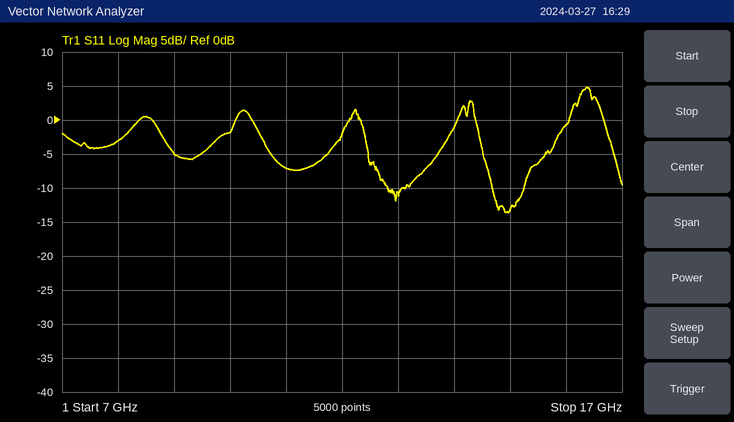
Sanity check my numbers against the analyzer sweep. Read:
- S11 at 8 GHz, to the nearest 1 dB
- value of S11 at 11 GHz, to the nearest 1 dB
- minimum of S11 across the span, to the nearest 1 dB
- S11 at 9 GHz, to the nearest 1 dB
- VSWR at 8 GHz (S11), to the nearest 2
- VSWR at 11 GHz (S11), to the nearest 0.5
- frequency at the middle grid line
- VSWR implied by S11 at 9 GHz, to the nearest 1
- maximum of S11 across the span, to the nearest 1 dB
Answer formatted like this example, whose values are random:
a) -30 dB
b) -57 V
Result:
a) -3 dB
b) -7 dB
c) -14 dB
d) -5 dB
e) 6
f) 2.5
g) 12 GHz
h) 4
i) 5 dB
